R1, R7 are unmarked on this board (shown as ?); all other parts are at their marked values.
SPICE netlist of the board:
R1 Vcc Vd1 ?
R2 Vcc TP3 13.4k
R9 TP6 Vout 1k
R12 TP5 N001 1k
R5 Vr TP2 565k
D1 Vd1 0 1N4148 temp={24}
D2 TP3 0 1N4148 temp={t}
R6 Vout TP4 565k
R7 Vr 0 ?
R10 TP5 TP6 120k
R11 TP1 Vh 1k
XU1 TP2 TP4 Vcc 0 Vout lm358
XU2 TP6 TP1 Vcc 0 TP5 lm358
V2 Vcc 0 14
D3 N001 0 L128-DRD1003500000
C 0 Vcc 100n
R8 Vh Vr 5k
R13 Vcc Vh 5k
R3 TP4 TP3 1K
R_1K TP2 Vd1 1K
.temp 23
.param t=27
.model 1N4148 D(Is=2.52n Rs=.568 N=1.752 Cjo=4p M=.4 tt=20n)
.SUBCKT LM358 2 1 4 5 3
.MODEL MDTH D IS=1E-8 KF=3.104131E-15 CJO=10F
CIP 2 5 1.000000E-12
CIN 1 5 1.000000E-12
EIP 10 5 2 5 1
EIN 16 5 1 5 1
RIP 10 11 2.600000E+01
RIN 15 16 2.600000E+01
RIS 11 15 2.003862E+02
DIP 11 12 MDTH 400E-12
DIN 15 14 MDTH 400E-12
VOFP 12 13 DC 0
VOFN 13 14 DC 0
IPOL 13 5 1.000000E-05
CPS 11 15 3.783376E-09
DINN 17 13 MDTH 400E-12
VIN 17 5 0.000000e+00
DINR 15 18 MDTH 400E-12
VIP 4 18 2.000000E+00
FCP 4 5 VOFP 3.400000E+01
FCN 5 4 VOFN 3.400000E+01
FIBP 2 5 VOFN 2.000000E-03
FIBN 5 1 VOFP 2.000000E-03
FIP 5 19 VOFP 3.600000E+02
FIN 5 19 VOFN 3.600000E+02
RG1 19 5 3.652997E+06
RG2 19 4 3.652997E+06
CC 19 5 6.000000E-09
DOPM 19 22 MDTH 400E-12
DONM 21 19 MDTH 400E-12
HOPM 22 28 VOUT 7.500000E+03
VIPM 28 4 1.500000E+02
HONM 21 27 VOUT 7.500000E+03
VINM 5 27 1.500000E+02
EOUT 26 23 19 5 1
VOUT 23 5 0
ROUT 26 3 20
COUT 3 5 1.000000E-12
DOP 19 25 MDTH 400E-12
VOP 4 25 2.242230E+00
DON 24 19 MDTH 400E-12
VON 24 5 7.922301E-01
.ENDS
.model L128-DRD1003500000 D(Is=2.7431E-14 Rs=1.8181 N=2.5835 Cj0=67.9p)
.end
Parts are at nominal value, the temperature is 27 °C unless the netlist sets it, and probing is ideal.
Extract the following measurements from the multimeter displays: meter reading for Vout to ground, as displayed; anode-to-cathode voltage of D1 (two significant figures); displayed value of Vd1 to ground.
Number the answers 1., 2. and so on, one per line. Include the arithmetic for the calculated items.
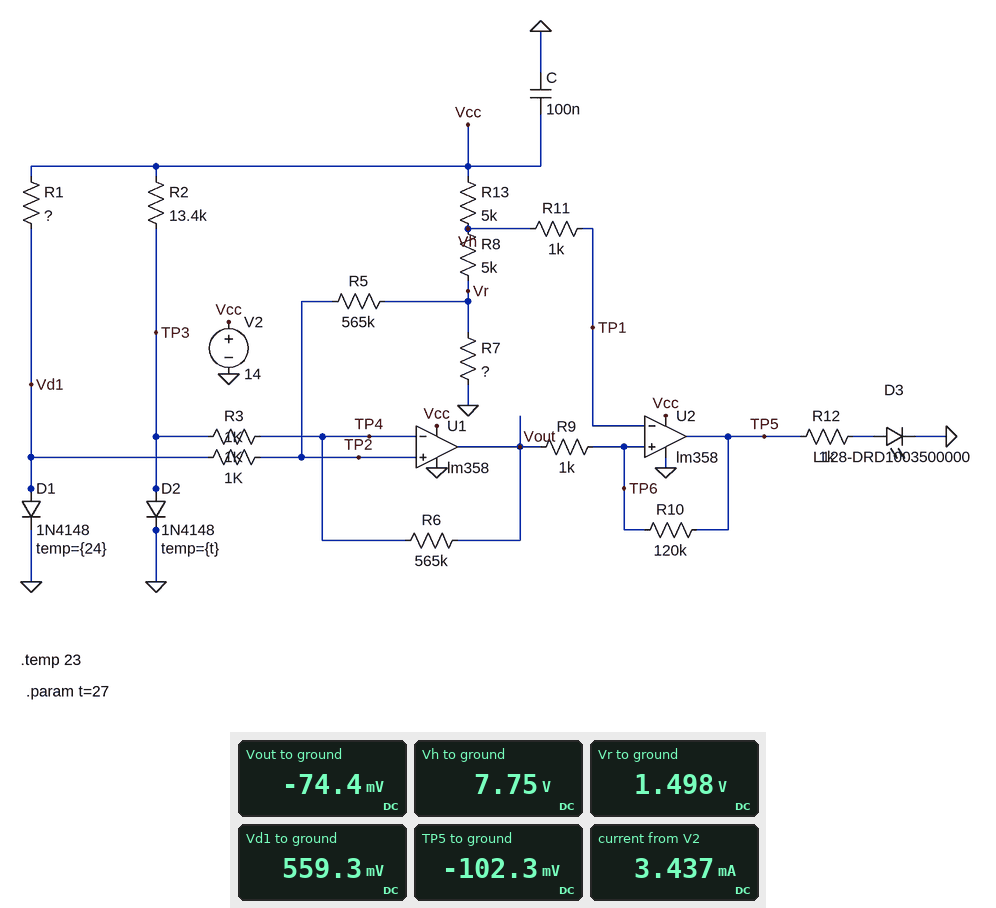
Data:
1. -74.4 mV
2. 559.3 mV = 560 mV
3. 559.3 mV
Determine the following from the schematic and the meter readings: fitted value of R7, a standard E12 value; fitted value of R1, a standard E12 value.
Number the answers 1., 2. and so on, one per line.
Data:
1. 1.2 kΩ
2. 27 kΩ
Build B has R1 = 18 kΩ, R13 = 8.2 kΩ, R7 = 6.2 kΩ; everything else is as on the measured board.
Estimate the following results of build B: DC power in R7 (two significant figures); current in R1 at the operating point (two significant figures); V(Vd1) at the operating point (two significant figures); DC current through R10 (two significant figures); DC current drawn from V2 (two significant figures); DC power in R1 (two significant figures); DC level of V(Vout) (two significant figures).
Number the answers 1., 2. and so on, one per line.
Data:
1. 3.2 mW
2. 750 µA
3. 580 mV
4. 5.6 µA
5. 3.2 mA
6. 10 mW
7. 570 mV
